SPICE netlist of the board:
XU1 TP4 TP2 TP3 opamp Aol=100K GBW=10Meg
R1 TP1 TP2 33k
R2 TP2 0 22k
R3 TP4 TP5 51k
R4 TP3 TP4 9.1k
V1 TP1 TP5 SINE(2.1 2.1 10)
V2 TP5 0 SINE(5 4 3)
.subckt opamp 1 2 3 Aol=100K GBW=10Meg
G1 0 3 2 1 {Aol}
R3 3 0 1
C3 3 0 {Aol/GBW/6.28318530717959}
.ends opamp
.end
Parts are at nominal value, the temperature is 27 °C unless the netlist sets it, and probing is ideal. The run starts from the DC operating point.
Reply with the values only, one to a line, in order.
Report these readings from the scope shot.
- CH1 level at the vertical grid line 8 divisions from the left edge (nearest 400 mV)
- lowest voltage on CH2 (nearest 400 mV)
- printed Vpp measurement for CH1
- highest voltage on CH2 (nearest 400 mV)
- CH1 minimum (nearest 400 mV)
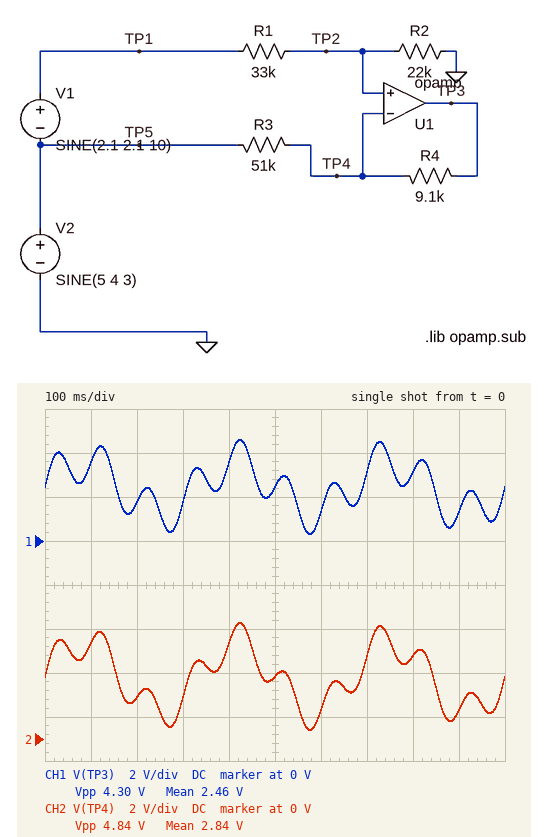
3.2 V
400 mV
4.30 V
5.2 V
400 mV
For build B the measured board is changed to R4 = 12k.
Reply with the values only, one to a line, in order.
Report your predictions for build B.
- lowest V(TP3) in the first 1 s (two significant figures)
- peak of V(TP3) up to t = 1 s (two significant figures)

270 mV
4.4 V
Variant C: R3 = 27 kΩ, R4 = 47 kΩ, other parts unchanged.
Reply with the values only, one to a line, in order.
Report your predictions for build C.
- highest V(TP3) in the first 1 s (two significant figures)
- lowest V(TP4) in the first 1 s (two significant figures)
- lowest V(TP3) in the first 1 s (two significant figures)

3.9 V
420 mV
-5.8 V
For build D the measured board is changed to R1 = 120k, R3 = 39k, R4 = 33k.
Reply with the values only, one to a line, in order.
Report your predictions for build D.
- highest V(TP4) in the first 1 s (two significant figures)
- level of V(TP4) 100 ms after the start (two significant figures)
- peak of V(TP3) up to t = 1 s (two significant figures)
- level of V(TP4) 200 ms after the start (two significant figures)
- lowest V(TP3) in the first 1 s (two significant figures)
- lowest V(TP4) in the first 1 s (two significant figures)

2.0 V
1.7 V
620 mV
740 mV
-5.0 V
160 mV
